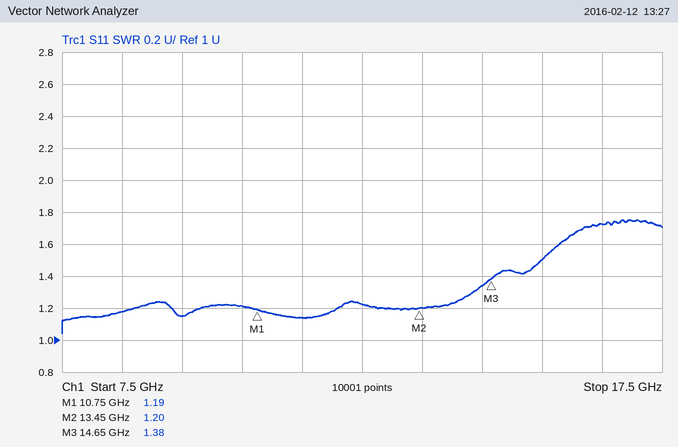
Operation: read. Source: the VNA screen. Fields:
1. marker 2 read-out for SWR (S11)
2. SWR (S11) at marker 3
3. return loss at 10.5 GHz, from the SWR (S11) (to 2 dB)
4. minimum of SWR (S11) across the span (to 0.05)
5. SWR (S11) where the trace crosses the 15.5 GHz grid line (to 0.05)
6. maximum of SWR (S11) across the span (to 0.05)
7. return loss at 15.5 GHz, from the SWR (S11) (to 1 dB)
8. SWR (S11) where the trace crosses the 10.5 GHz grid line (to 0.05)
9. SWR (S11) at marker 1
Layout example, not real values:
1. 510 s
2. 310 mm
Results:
1. 1.20
2. 1.38
3. 20 dB
4. 1.05
5. 1.50
6. 1.75
7. 14 dB
8. 1.20
9. 1.19
